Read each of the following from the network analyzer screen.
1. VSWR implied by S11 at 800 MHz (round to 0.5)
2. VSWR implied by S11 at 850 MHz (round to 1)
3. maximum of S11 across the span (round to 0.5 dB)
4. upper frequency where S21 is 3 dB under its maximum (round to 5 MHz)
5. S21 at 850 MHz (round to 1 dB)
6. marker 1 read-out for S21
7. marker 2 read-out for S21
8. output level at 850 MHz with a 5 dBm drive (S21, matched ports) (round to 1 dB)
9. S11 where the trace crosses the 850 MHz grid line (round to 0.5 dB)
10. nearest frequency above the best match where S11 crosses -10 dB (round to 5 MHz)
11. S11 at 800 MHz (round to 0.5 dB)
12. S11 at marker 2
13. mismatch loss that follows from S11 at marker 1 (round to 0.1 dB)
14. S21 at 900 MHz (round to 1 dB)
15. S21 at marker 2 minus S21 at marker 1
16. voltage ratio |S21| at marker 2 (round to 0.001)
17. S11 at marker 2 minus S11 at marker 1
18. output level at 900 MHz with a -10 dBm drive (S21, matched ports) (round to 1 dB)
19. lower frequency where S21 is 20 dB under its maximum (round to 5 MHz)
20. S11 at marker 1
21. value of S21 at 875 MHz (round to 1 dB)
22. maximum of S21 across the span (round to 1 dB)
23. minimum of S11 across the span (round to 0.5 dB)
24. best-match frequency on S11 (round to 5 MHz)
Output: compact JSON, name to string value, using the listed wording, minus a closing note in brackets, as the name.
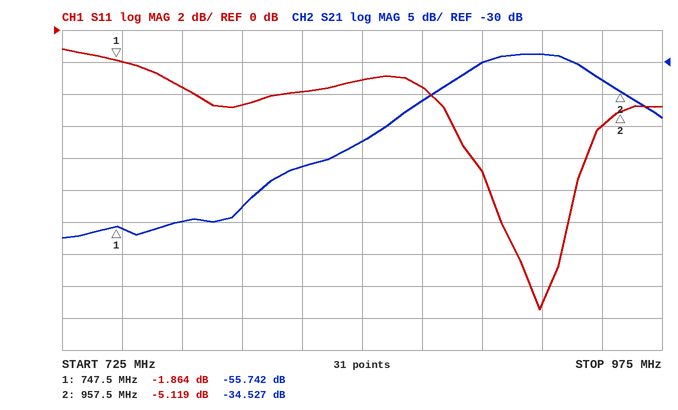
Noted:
{"VSWR implied by S11 at 800 MHz": "4.0", "VSWR implied by S11 at 850 MHz": "6", "maximum of S11 across the span": "-1.0 dB", "upper frequency where S21 is 3 dB under its maximum": "945 MHz", "S21 at 850 MHz": "-42 dB", "marker 1 read-out for S21": "-55.742 dB", "marker 2 read-out for S21": "-34.527 dB", "output level at 850 MHz with a 5 dBm drive (S21, matched ports)": "-37 dBm", "S11 where the trace crosses the 850 MHz grid line": "-3.0 dB", "nearest frequency above the best match where S11 crosses -10 dB": "940 MHz", "S11 at 800 MHz": "-4.5 dB", "S11 at marker 2": "-5.119 dB", "mismatch loss that follows from S11 at marker 1": "4.6 dB", "S21 at 900 MHz": "-30 dB", "S21 at marker 2 minus S21 at marker 1": "21.215 dB", "voltage ratio |S21| at marker 2": "0.019", "S11 at marker 2 minus S11 at marker 1": "-3.255 dB", "output level at 900 MHz with a -10 dBm drive (S21, matched ports)": "-40 dBm", "lower frequency where S21 is 20 dB under its maximum": "810 MHz", "S11 at marker 1": "-1.864 dB", "value of S21 at 875 MHz": "-36 dB", "maximum of S21 across the span": "-29 dB", "minimum of S11 across the span": "-17.5 dB", "best-match frequency on S11": "925 MHz"}
